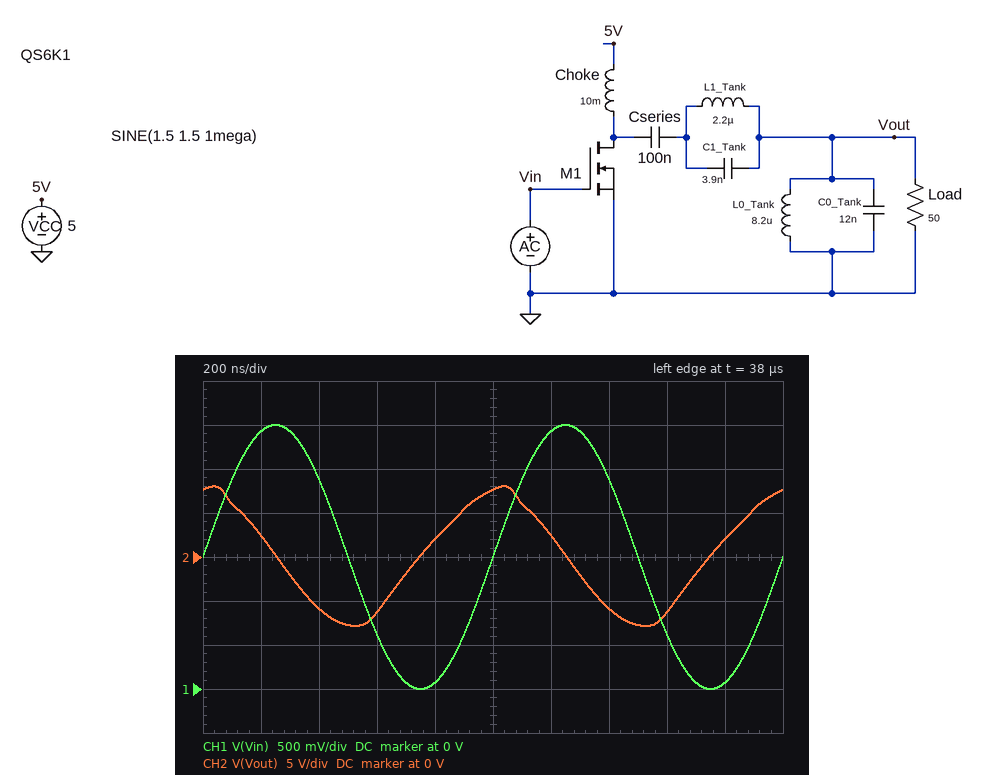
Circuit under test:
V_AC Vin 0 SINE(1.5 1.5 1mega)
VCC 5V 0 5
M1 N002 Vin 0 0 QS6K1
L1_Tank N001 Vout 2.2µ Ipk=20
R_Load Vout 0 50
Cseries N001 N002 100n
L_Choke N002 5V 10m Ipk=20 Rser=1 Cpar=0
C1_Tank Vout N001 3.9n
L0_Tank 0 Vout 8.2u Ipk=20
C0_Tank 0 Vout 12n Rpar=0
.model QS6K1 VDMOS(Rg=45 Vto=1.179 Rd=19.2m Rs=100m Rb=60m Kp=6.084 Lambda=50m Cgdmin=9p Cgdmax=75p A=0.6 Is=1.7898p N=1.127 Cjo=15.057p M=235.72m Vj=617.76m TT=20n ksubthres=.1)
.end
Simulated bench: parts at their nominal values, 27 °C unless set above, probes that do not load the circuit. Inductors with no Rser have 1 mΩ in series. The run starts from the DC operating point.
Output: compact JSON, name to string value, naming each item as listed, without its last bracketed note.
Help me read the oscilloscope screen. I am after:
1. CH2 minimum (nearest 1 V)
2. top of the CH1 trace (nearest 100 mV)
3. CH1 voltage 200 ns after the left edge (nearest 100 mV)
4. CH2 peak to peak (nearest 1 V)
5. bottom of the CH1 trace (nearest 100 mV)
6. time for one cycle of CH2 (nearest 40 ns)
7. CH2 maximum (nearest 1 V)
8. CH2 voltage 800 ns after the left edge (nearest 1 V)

{"CH2 minimum": "-8 V", "top of the CH1 trace": "3.0 V", "CH1 voltage 200 ns after the left edge": "2.9 V", "CH2 peak to peak": "16 V", "bottom of the CH1 trace": "0 V", "time for one cycle of CH2": "1.00 µs", "CH2 maximum": "8 V", "CH2 voltage 800 ns after the left edge": "2 V"}
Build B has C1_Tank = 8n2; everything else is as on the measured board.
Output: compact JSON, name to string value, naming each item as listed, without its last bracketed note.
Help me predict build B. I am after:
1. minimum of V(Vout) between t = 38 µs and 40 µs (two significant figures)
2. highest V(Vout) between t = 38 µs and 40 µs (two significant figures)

{"minimum of V(Vout) between t = 38 µs and 40 µs": "-22 V", "highest V(Vout) between t = 38 µs and 40 µs": "25 V"}
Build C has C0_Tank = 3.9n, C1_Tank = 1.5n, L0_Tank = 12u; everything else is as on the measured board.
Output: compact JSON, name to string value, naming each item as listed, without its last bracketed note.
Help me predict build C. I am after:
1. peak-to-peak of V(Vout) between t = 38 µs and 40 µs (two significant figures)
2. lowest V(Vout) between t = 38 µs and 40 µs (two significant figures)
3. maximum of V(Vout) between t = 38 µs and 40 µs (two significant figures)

{"peak-to-peak of V(Vout) between t = 38 µs and 40 µs": "33 V", "lowest V(Vout) between t = 38 µs and 40 µs": "-18 V", "maximum of V(Vout) between t = 38 µs and 40 µs": "15 V"}
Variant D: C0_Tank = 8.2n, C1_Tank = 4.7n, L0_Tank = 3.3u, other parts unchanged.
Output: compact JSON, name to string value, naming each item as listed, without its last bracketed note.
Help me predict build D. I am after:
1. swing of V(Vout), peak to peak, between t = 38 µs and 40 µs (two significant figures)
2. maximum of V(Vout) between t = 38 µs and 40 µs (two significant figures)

{"swing of V(Vout), peak to peak, between t = 38 µs and 40 µs": "38 V", "maximum of V(Vout) between t = 38 µs and 40 µs": "19 V"}
